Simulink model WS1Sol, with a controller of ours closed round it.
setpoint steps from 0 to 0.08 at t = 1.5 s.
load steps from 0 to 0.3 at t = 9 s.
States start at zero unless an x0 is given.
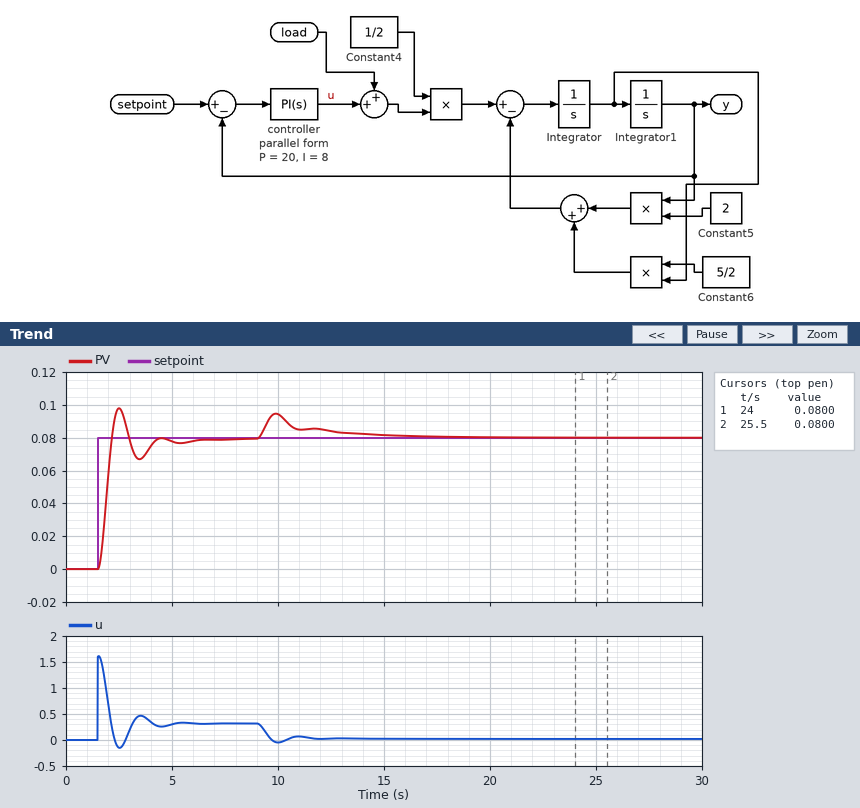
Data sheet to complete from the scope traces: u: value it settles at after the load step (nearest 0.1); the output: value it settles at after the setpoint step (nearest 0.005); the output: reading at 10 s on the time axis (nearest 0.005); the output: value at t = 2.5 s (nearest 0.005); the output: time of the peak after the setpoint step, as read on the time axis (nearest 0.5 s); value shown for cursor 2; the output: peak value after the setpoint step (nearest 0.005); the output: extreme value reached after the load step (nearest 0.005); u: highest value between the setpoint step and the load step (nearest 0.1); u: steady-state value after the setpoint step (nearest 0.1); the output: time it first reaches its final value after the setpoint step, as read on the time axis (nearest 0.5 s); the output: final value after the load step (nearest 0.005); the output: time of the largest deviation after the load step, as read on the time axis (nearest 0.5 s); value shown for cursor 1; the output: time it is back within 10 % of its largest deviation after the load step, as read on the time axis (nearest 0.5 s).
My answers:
0.0
0.080
0.095
0.100
2.5 s
0.0800
0.100
0.095
1.6
0.3
2.0 s
0.080
10.0 s
0.0800
15.0 s
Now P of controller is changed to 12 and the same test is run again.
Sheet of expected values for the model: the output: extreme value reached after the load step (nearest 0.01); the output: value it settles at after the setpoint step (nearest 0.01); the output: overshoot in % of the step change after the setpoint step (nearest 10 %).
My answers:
0.10
0.08
20 %
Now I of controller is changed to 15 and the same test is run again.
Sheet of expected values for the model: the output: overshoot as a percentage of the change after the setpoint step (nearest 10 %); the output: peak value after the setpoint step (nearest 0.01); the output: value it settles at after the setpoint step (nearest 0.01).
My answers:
30 %
0.11
0.08
